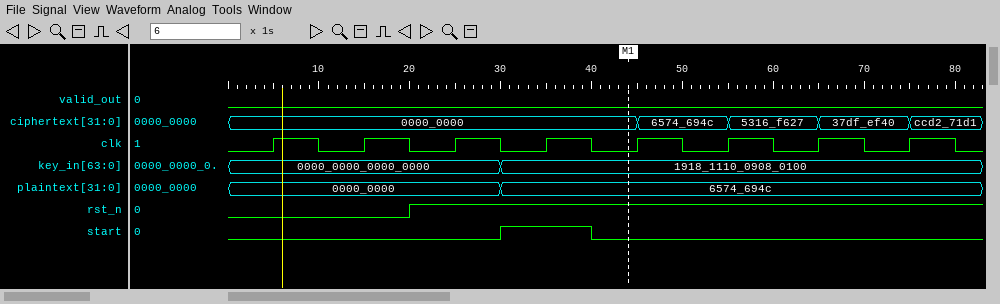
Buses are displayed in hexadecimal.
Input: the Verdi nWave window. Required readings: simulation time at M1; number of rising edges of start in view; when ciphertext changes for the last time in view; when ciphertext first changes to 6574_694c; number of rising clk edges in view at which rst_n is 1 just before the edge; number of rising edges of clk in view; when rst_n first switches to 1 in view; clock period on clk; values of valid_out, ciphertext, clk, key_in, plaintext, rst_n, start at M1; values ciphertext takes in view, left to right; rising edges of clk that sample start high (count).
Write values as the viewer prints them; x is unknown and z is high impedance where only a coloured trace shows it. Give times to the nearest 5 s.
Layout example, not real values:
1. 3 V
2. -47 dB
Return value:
1. 45 s
2. 1
3. 75 s
4. 45 s
5. 6
6. 8
7. 20 s
8. 10 s
9. valid_out=0, ciphertext=0000_0000, clk=0, key_in=1918_1110_0908_0100, plaintext=6574_694c, rst_n=1, start=0
10. 0000_0000, 6574_694c, 5316_f627, 37df_ef40, ccd2_71d1
11. 1
